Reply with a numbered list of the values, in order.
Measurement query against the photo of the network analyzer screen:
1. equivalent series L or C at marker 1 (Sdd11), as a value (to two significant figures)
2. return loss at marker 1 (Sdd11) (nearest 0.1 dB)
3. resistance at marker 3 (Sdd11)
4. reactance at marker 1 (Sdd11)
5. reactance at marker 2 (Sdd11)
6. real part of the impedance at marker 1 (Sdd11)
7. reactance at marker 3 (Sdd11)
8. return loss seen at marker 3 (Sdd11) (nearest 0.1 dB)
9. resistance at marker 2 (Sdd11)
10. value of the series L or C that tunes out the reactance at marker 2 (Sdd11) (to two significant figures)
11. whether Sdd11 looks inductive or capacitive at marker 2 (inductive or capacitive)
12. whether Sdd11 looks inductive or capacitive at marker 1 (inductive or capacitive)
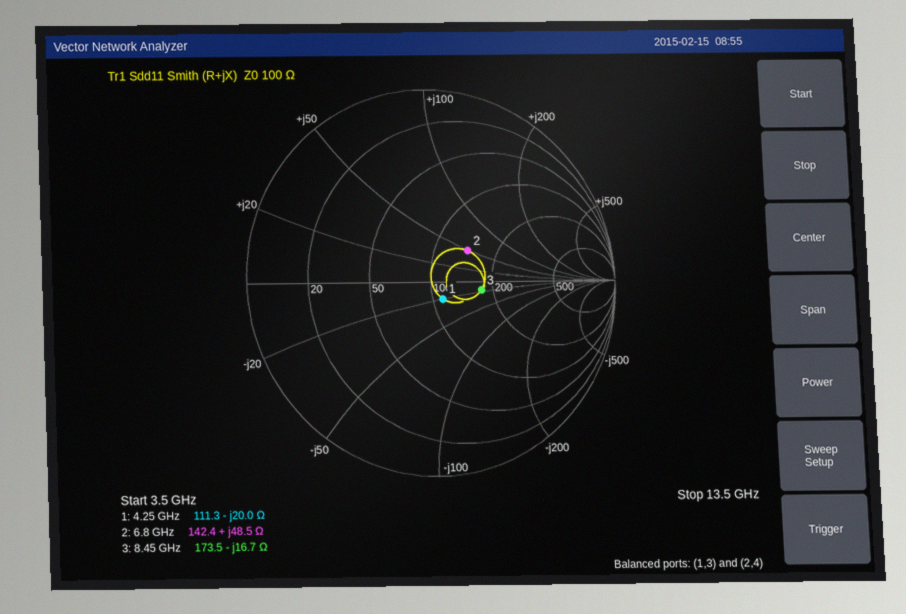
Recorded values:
1. 1.9 pF
2. 19.3 dB
3. 173.5 Ω
4. -20.0 Ω
5. +48.5 Ω
6. 111.3 Ω
7. -16.7 Ω
8. 11.2 dB
9. 142.4 Ω
10. 480 fF
11. inductive
12. capacitive
